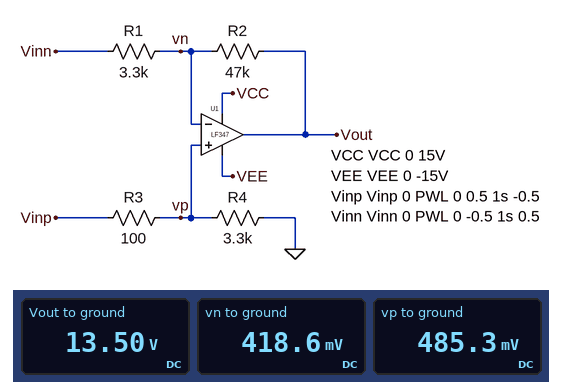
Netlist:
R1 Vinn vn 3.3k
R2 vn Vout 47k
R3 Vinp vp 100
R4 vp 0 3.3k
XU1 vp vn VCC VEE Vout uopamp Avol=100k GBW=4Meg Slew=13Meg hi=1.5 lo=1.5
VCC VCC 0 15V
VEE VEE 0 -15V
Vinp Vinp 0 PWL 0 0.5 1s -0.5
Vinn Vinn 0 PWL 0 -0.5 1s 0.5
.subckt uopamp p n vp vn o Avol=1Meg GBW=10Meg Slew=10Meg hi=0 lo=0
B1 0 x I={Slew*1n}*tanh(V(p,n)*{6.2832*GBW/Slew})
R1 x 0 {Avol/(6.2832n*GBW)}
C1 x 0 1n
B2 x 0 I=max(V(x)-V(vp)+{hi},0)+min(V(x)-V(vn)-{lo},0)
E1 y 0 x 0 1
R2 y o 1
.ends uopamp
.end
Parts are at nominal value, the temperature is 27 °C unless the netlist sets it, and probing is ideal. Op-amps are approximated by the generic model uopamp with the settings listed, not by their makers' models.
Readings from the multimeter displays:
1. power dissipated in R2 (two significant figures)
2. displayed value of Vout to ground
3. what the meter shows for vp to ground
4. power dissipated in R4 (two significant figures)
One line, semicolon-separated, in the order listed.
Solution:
3.6 mW; 13.50 V; 485.3 mV; 71 µW
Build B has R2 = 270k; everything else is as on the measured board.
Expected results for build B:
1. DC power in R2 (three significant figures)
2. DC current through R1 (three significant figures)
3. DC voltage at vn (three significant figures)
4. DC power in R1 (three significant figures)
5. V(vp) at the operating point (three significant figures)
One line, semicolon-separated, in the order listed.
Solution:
710 µW; 51.3 µA; -331 mV; 8.67 µW; 485 mV
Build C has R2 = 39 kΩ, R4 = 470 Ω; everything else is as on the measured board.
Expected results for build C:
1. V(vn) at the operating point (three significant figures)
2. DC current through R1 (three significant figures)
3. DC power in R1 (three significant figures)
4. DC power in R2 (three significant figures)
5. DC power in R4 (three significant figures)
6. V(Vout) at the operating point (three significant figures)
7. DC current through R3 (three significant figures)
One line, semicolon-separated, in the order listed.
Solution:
412 mV; 276 µA; 252 µW; 2.98 mW; 362 µW; 11.2 V; 877 µA
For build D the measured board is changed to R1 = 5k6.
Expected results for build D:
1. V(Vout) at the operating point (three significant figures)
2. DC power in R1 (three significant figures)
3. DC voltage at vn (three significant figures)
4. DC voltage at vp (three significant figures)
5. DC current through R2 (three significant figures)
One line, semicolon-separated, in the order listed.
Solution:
8.75 V; 173 µW; 485 mV; 485 mV; 176 µA
